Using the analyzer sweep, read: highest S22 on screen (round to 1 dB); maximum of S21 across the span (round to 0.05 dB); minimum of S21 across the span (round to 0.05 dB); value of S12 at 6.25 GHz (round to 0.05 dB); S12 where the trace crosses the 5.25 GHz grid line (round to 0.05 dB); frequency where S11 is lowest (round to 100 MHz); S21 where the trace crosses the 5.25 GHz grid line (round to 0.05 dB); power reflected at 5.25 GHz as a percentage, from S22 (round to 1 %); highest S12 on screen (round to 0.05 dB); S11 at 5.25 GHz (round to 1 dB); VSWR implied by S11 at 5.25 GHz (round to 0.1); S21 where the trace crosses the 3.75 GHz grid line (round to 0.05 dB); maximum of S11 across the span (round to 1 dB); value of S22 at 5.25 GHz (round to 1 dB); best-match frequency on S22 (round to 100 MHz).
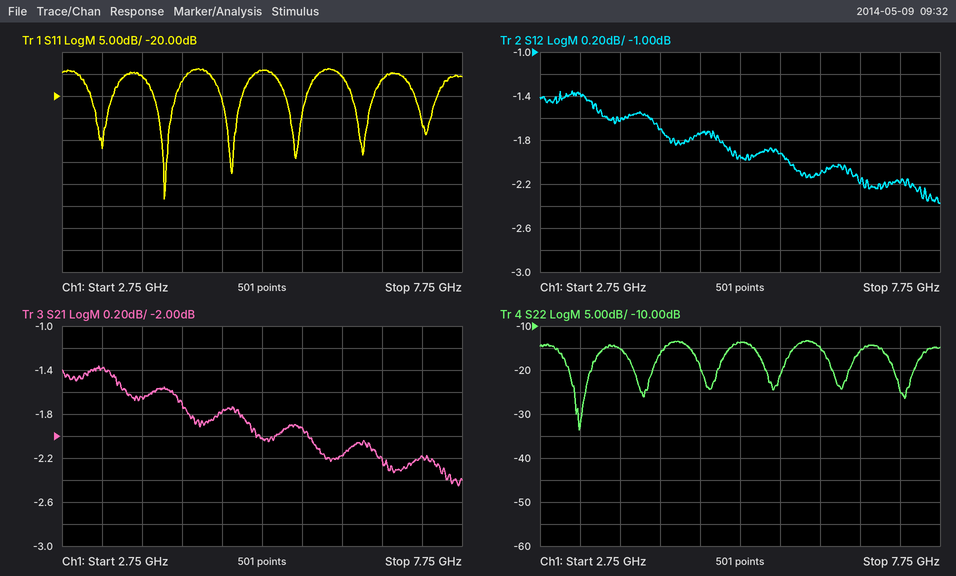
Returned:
-13 dB
-1.35 dB
-2.45 dB
-2.10 dB
-1.95 dB
4.0 GHz
-2.00 dB
4 %
-1.35 dB
-14 dB
1.5
-1.65 dB
-14 dB
-14 dB
3.2 GHz
